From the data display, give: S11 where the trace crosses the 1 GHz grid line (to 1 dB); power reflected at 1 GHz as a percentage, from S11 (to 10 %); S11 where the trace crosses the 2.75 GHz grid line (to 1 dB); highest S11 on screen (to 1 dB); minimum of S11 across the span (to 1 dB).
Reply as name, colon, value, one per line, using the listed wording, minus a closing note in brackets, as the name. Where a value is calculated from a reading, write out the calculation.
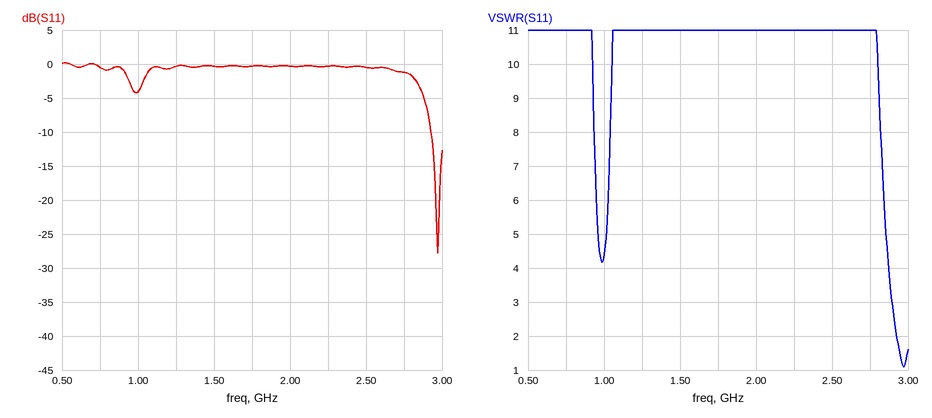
S11 where the trace crosses the 1 GHz grid line: -4 dB
power reflected at 1 GHz as a percentage, from S11: 10^(-4/10) ≈ 40 %
S11 where the trace crosses the 2.75 GHz grid line: -1 dB
highest S11 on screen: 0 dB
minimum of S11 across the span: -28 dB
